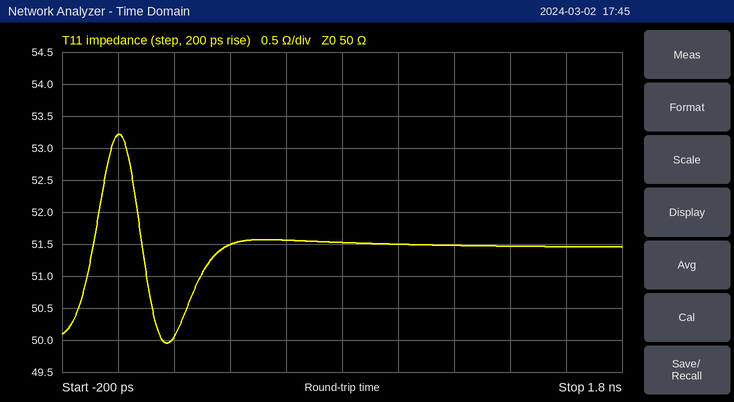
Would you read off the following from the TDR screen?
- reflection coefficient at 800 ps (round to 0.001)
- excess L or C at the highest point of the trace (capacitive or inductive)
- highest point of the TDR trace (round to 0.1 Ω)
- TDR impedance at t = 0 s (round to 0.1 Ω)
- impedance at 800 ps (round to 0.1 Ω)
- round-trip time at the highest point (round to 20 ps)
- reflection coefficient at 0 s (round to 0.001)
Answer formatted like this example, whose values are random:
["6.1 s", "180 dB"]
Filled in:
["+0.015", "inductive", "53.2 Ω", "53.2 Ω", "51.5 Ω", "0 ps", "+0.031"]
